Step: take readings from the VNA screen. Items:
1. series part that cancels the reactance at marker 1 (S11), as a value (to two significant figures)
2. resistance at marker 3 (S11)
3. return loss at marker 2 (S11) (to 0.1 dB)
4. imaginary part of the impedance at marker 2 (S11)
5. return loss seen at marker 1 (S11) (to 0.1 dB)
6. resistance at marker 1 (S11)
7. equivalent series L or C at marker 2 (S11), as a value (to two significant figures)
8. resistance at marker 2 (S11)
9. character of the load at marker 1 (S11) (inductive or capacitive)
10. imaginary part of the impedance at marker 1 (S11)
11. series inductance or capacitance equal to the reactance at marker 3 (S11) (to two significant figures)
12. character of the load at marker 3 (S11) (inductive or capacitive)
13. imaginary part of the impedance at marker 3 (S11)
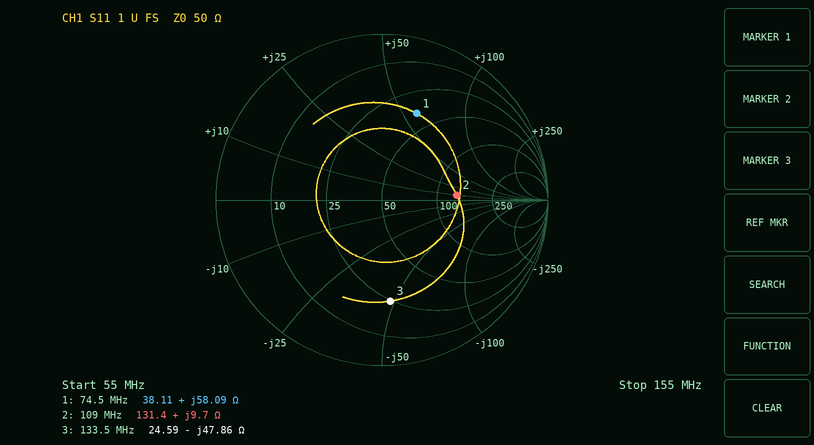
37 pF
24.59 Ω
6.9 dB
+9.7 Ω
5.0 dB
38.11 Ω
14 nH
131.4 Ω
inductive
+58.09 Ω
25 pF
capacitive
-47.86 Ω
